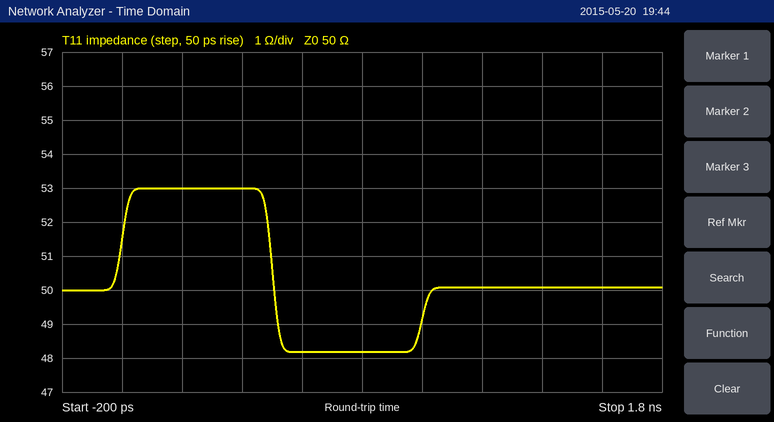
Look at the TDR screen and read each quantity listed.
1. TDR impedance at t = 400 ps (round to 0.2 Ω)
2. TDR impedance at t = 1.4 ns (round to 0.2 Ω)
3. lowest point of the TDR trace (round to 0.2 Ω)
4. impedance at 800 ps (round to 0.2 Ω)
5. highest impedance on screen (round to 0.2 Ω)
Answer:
53.0 Ω
50.0 Ω
48.2 Ω
48.2 Ω
53.0 Ω
